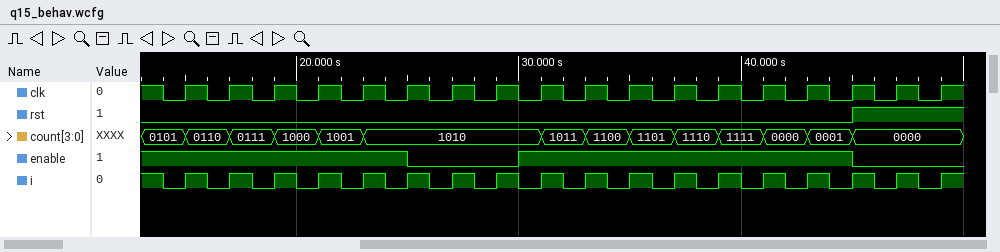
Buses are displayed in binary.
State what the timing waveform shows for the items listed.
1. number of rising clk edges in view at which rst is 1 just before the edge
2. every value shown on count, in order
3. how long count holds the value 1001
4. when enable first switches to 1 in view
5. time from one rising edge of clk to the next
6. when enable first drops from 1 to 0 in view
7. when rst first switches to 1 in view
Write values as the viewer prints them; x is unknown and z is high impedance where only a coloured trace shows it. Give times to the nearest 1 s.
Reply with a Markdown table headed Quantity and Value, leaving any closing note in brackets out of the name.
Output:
| Quantity | Value |
|---|---|
| number of rising clk edges in view at which rst is 1 just before the edge | 2 |
| every value shown on count, in order | 0101, 0110, 0111, 1000, 1001, 1010, 1011, 1100, 1101, 1110, 1111, 0000, 0001, 0000 |
| how long count holds the value 1001 | 2 s |
| when enable first switches to 1 in view | 30 s |
| time from one rising edge of clk to the next | 2 s |
| when enable first drops from 1 to 0 in view | 25 s |
| when rst first switches to 1 in view | 45 s |
